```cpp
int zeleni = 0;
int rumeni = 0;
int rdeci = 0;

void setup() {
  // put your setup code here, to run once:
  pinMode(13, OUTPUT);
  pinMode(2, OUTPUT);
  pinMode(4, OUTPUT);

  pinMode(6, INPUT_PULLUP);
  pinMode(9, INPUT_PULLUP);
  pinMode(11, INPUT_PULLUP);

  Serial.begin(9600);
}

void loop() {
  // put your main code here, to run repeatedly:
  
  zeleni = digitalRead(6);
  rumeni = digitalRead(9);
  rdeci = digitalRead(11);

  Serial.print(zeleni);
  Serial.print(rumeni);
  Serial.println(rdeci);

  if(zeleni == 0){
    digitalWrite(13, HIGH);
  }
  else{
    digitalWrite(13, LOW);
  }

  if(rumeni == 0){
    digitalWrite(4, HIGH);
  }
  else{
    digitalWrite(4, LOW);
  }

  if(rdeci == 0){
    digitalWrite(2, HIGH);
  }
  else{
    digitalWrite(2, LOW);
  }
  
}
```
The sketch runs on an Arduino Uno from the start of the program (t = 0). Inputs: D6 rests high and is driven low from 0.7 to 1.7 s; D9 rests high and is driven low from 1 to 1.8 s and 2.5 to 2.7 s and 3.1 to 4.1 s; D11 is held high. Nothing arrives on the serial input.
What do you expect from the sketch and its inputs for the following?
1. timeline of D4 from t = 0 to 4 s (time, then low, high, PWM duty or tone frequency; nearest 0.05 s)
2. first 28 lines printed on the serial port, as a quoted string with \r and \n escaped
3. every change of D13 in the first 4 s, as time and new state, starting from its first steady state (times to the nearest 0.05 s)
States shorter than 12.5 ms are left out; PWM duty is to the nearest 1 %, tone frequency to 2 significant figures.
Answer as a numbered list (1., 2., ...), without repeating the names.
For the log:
1. 0 s low; 1 s high; 1.8 s low; 2.5 s high; 2.7 s low; 3.1 s high
2. "111\r\n111\r\n111\r\n111\r\n111\r\n111\r\n111\r\n111\r\n111\r\n111\r\n111\r\n111\r\n111\r\n111\r\n111\r\n111\r\n111\r\n111\r\n111\r\n111\r\n111\r\n111\r\n111\r\n111\r\n111\r\n111\r\n111\r\n111\r\n"
3. 0 s low; 0.7 s high; 1.7 s low
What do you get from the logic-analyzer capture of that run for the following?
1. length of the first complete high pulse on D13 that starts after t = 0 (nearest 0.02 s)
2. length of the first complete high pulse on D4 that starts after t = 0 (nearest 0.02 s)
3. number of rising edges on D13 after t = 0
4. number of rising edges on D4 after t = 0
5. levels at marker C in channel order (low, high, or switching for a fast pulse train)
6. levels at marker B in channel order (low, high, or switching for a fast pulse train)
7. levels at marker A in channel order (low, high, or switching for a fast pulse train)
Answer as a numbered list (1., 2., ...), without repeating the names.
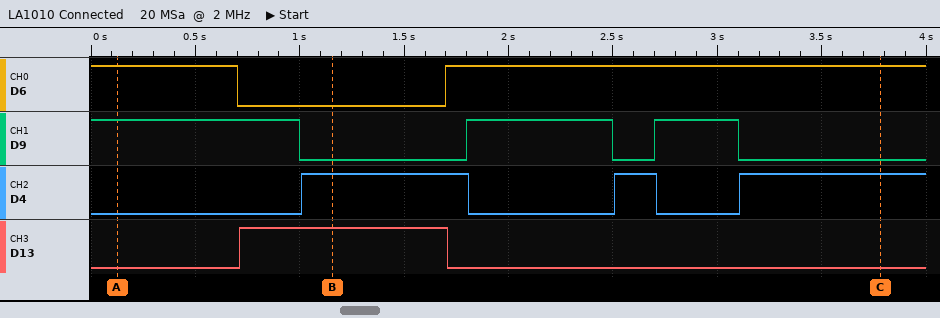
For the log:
1. 1.00 s
2. 0.80 s
3. 1
4. 3
5. D6 high, D9 low, D4 high, D13 low
6. D6 low, D9 low, D4 high, D13 high
7. D6 high, D9 high, D4 low, D13 low
